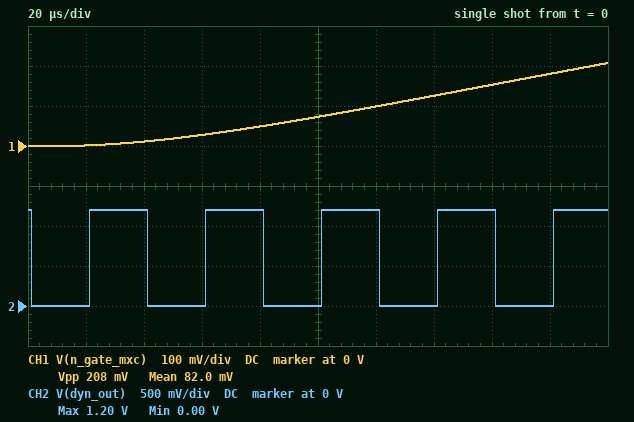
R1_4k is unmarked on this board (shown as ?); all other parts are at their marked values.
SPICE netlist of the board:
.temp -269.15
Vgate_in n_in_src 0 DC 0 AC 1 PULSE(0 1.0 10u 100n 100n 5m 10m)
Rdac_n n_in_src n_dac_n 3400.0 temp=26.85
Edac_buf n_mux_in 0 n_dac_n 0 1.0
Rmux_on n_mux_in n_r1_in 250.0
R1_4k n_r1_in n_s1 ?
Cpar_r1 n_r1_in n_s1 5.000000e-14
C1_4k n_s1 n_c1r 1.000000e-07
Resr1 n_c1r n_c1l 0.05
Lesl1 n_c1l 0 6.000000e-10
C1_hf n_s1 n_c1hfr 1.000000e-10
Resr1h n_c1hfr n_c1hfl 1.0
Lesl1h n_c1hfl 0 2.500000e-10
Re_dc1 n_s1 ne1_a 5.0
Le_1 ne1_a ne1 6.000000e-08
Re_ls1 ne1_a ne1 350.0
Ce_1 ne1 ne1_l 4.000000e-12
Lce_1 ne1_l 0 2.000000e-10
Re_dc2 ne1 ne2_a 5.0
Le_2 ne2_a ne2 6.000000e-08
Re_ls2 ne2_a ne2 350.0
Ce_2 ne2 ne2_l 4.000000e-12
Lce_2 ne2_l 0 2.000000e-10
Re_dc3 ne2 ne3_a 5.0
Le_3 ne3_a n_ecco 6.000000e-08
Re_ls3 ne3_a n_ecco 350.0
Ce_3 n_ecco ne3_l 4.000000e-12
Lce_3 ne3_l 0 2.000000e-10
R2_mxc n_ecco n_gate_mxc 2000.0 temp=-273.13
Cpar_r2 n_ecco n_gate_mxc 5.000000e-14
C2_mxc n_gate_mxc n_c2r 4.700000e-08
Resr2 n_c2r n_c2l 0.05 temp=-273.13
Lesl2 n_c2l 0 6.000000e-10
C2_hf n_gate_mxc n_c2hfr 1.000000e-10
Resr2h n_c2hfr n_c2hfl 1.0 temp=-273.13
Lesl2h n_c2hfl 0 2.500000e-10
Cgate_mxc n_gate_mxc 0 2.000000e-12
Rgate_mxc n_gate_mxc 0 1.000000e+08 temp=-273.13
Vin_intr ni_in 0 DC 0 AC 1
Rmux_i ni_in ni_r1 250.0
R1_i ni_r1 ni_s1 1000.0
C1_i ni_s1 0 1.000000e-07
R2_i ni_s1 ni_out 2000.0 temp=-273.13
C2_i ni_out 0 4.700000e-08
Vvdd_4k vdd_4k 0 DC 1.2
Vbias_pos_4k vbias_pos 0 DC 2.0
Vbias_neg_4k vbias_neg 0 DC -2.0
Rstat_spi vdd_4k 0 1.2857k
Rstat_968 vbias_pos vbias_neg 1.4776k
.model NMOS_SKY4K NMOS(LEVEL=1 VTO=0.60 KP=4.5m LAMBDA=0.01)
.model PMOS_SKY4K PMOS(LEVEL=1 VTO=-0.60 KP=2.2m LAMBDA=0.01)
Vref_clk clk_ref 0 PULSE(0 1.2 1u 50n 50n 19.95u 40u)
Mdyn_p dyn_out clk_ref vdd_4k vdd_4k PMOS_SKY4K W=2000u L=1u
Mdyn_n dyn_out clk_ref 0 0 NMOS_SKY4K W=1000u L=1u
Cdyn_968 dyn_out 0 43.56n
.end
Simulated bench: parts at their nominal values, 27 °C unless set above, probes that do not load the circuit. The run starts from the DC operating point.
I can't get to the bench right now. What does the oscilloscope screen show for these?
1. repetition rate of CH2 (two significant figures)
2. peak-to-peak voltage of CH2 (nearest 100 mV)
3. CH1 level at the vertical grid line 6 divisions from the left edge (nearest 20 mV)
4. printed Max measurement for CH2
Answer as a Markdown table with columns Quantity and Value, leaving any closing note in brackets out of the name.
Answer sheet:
| Quantity | Value |
|---|---|
| repetition rate of CH2 | 25 kHz |
| peak-to-peak voltage of CH2 | 1.2 V |
| CH1 level at the vertical grid line 6 divisions from the left edge | 100 mV |
| printed Max measurement for CH2 | 1.20 V |
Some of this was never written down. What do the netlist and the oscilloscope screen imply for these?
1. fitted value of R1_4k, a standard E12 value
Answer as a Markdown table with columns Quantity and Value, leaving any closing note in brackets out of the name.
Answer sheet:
| Quantity | Value |
|---|---|
| fitted value of R1_4k, a standard E12 value | 3.3 kΩ |
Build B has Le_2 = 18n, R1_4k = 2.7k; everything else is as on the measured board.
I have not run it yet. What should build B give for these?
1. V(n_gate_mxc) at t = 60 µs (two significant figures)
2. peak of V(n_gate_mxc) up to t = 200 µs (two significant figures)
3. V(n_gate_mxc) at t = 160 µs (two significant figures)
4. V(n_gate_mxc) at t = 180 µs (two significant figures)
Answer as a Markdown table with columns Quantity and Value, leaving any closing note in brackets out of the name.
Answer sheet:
| Quantity | Value |
|---|---|
| V(n_gate_mxc) at t = 60 µs | 33 mV |
| peak of V(n_gate_mxc) up to t = 200 µs | 240 mV |
| V(n_gate_mxc) at t = 160 µs | 180 mV |
| V(n_gate_mxc) at t = 180 µs | 210 mV |
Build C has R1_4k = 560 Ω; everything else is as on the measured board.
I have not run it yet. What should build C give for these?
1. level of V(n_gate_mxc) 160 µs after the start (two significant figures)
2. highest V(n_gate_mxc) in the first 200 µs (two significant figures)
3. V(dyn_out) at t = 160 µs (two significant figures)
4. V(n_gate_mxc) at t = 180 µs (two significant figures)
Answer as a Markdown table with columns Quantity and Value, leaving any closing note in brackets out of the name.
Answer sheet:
| Quantity | Value |
|---|---|
| level of V(n_gate_mxc) 160 µs after the start | 450 mV |
| highest V(n_gate_mxc) in the first 200 µs | 560 mV |
| V(dyn_out) at t = 160 µs | 1.2 V |
| V(n_gate_mxc) at t = 180 µs | 510 mV |
